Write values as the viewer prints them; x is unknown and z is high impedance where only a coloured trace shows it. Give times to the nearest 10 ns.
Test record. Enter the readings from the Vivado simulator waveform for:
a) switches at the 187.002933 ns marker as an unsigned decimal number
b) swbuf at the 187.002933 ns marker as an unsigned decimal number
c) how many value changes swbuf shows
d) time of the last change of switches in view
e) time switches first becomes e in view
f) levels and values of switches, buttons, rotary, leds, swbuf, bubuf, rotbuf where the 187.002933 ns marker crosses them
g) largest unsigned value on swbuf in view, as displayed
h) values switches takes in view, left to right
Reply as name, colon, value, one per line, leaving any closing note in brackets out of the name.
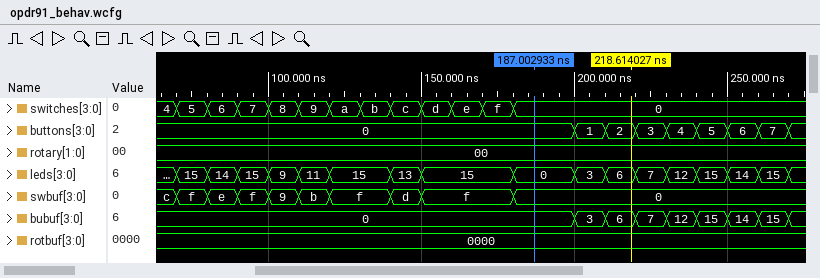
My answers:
switches at the 187.002933 ns marker as an unsigned decimal number: 0
swbuf at the 187.002933 ns marker as an unsigned decimal number: 0
how many value changes swbuf shows: 9
time of the last change of switches in view: 180 ns
time switches first becomes e in view: 160 ns
levels and values of switches, buttons, rotary, leds, swbuf, bubuf, rotbuf where the 187.002933 ns marker crosses them: switches=0, buttons=0, rotary=00, leds=0, swbuf=0, bubuf=0, rotbuf=0000
largest unsigned value on swbuf in view, as displayed: f
values switches takes in view, left to right: 4, 5, 6, 7, 8, 9, a, b, c, d, e, f, 0
